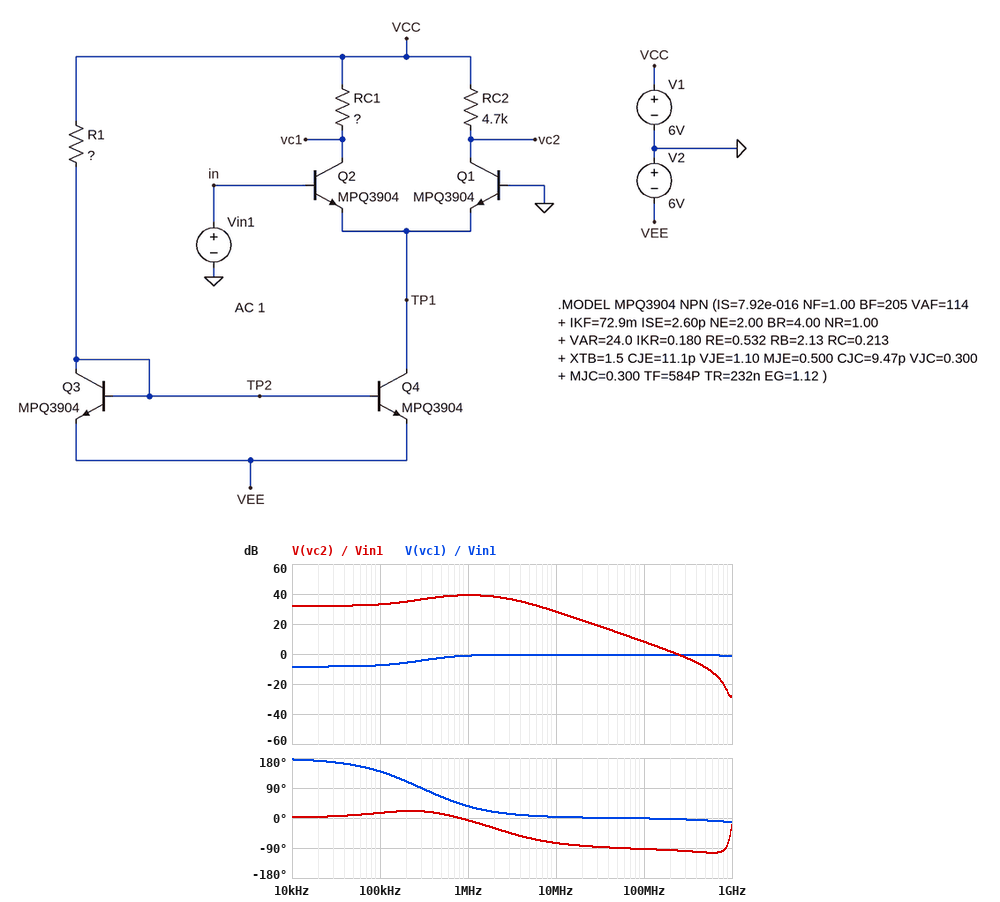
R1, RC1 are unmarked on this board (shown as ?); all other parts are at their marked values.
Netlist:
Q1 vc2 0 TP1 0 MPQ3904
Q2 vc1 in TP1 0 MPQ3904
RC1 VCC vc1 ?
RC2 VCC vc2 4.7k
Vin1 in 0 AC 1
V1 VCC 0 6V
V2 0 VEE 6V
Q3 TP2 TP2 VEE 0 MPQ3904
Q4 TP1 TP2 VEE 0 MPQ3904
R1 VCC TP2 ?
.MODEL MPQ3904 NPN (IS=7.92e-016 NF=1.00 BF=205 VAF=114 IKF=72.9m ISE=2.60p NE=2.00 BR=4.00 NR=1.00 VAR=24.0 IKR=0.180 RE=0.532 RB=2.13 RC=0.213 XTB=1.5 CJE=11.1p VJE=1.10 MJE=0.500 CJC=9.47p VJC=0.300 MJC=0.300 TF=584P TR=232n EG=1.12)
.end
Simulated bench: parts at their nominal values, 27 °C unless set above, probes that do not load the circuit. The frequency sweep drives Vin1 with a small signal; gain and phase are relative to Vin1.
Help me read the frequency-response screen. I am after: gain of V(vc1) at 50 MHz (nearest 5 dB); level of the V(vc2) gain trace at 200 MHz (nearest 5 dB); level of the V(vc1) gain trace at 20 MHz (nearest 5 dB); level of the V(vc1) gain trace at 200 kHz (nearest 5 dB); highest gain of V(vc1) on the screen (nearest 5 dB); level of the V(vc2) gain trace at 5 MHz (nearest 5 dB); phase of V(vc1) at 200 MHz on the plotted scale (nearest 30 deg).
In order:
0 dB
0 dB
0 dB
-5 dB
0 dB
35 dB
0 deg
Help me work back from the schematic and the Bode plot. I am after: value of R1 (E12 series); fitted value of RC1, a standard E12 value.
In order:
5.6 kΩ
12 kΩ
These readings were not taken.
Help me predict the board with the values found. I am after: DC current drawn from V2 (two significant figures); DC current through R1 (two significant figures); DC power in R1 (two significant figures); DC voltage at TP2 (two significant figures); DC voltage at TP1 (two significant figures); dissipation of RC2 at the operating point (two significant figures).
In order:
4.1 mA
2.0 mA
23 mW
-5.3 V
-730 mV
8.2 mW
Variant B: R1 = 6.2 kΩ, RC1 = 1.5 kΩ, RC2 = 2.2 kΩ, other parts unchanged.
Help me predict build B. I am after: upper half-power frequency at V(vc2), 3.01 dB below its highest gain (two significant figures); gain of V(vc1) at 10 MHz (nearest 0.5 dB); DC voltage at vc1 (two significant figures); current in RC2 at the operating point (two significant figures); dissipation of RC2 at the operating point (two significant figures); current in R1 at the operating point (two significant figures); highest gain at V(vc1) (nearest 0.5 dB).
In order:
16 MHz
27.5 dB
4.6 V
920 µA
1.9 mW
1.8 mA
28.0 dB
